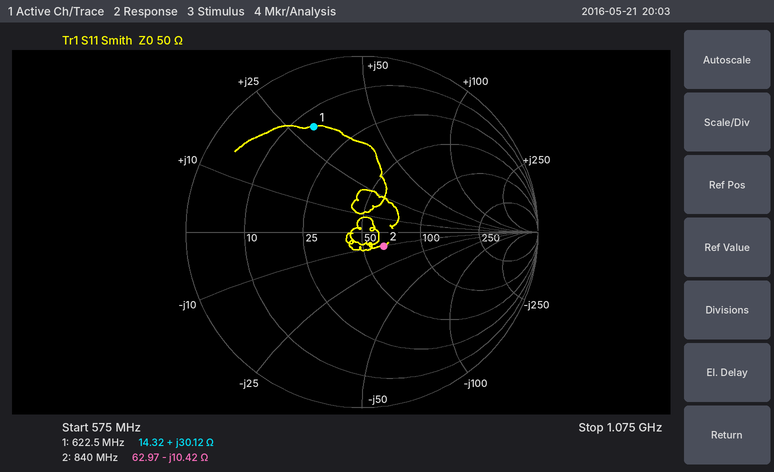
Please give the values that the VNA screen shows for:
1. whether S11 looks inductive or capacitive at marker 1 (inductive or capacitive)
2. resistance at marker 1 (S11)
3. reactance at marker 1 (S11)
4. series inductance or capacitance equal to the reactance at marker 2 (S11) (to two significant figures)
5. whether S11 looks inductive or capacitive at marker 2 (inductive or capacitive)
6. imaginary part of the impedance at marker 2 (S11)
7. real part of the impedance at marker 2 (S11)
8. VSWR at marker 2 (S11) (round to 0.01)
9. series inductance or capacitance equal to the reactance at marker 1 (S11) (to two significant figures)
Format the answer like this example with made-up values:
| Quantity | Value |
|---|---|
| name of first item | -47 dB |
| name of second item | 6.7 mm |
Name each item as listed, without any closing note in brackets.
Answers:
| Quantity | Value |
|---|---|
| whether S11 looks inductive or capacitive at marker 1 | inductive |
| resistance at marker 1 | 14.32 Ω |
| reactance at marker 1 | +30.12 Ω |
| series inductance or capacitance equal to the reactance at marker 2 (S11) | 18 pF |
| whether S11 looks inductive or capacitive at marker 2 | capacitive |
| imaginary part of the impedance at marker 2 | -10.42 Ω |
| real part of the impedance at marker 2 | 62.97 Ω |
| VSWR at marker 2 (S11) | 1.34 |
| series inductance or capacitance equal to the reactance at marker 1 (S11) | 7.7 nH |
